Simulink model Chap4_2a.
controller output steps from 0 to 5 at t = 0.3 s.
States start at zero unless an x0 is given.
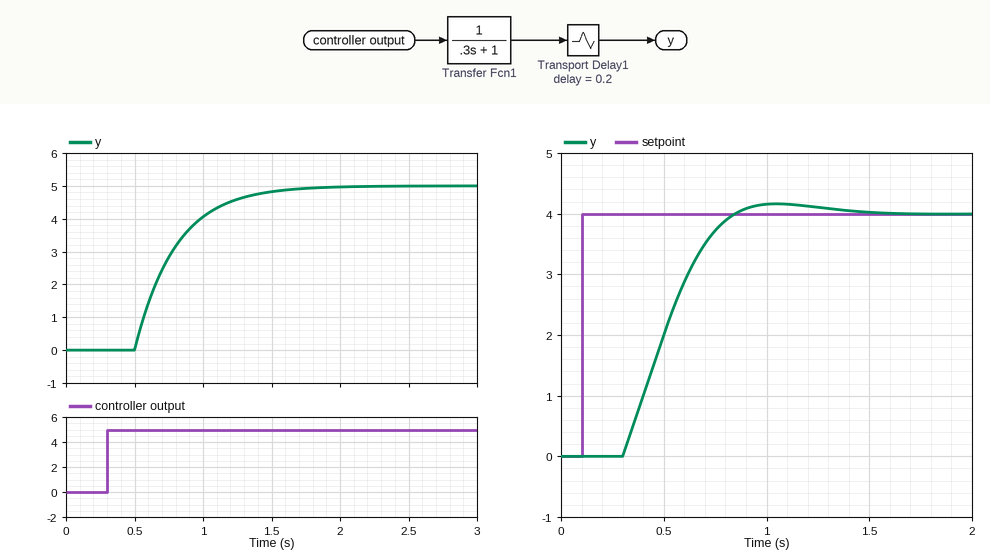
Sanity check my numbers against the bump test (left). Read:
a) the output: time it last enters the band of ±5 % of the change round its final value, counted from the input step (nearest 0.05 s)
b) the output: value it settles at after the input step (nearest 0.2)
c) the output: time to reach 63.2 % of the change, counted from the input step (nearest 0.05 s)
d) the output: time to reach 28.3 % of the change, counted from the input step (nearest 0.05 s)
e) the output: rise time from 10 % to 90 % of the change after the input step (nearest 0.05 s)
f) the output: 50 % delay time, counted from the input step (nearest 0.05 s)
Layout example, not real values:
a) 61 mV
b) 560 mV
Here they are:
a) 1.10 s
b) 5.0
c) 0.50 s
d) 0.30 s
e) 0.65 s
f) 0.40 s
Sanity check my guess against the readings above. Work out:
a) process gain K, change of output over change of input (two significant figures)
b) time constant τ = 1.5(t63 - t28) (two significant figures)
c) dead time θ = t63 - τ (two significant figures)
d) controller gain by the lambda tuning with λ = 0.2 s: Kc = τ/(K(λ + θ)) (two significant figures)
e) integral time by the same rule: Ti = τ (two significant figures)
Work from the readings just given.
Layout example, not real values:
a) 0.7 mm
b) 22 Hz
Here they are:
a) 1.0
b) 0.30 s
c) 0.20 s
d) 0.75
e) 0.30 s
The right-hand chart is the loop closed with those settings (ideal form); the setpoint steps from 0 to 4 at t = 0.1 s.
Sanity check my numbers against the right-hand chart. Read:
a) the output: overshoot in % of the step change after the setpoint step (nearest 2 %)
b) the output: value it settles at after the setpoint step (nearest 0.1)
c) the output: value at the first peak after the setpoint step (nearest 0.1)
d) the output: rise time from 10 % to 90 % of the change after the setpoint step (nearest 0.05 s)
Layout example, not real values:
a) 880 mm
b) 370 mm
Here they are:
a) 4 %
b) 4.0
c) 4.2
d) 0.40 s
